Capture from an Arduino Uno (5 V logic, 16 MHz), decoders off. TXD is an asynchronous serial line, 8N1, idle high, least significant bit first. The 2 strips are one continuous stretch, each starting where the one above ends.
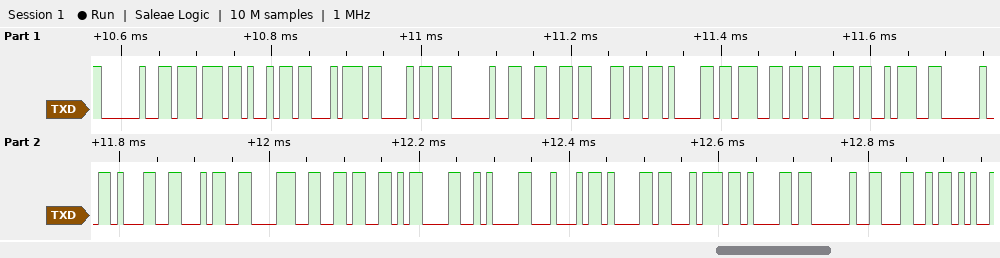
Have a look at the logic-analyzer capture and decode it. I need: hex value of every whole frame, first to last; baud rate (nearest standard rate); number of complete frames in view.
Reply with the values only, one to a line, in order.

20 77 69 74 68 20 66 6C 61 67 73 3A 20 31 34 38 36 0D 0A 44 61 74 61 20 4C
115200 baud
25
